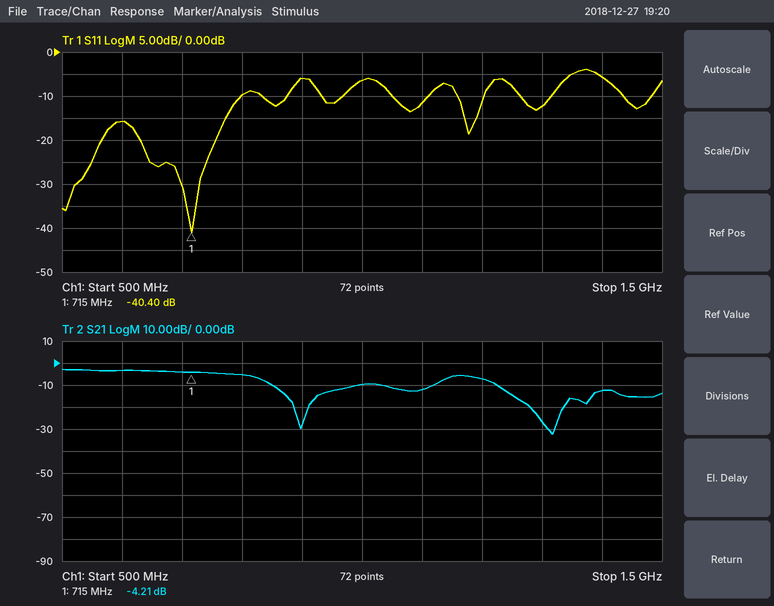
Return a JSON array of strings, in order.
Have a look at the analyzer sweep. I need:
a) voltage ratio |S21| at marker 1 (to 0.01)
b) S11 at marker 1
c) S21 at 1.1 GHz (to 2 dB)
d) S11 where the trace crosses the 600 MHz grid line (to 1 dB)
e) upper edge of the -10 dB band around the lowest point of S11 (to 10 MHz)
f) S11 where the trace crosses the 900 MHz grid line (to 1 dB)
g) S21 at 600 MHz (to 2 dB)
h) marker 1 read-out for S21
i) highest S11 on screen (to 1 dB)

["0.62", "-40.40 dB", "-12 dB", "-16 dB", "800 MHz", "-6 dB", "-4 dB", "-4.21 dB", "-4 dB"]
